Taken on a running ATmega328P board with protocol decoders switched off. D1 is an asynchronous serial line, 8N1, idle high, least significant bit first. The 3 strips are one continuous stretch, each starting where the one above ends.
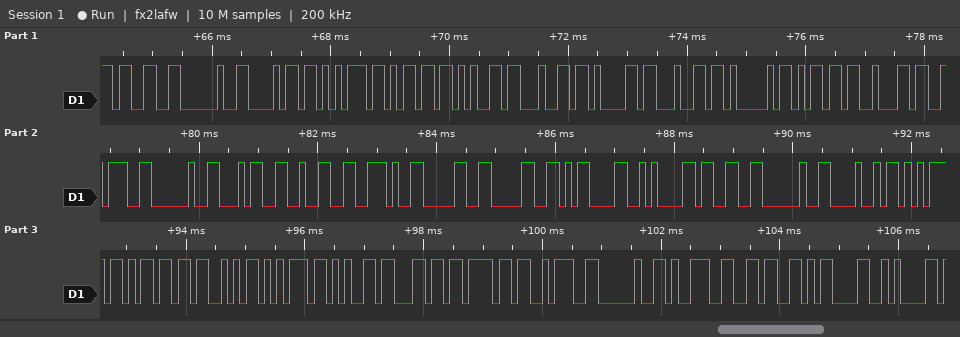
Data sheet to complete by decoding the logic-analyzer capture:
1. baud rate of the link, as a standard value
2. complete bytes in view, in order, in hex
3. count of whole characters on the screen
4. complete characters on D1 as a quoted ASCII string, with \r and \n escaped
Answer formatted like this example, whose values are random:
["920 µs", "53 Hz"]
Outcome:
["9600 baud", "33 20 68 75 6D 65 64 61 64 41 6D 62 3A 20 34 32 2E 30 30 0D 0A 33 20 48 75 6D 53 75 65 6C 6F 3A 20 39 36 0D 0A", "37", "\"3 humedadAmb: 42.00\\r\\n3 HumSuelo: 96\\r\\n\""]
